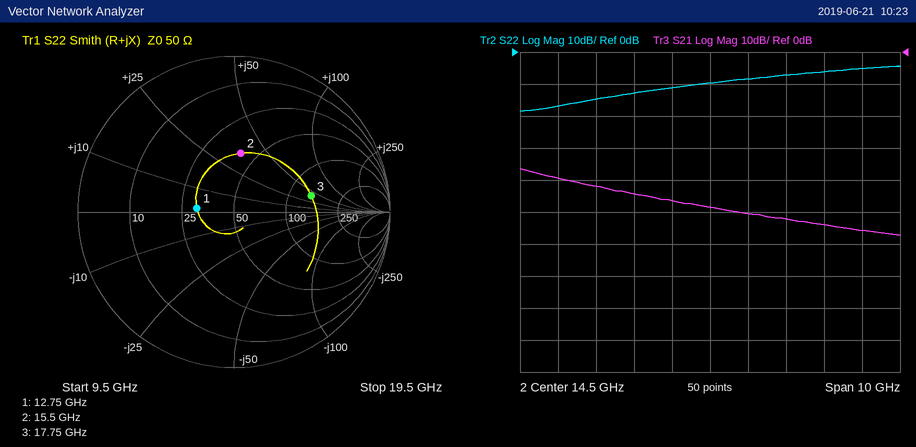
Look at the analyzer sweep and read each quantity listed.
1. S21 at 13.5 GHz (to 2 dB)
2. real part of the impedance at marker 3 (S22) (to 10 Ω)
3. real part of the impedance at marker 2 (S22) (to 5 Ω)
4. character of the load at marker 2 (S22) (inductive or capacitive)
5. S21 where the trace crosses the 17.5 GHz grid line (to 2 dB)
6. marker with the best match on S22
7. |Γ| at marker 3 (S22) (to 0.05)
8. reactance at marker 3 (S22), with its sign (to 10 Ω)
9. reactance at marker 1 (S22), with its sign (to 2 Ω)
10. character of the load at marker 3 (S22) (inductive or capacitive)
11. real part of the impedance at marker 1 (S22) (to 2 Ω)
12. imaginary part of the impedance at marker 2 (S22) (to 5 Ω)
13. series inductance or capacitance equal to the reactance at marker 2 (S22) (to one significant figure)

-46 dB
140 Ω
40 Ω
inductive
-54 dB
marker 1
0.50
+40 Ω
+2 Ω
inductive
30 Ω
+35 Ω
400 pH
